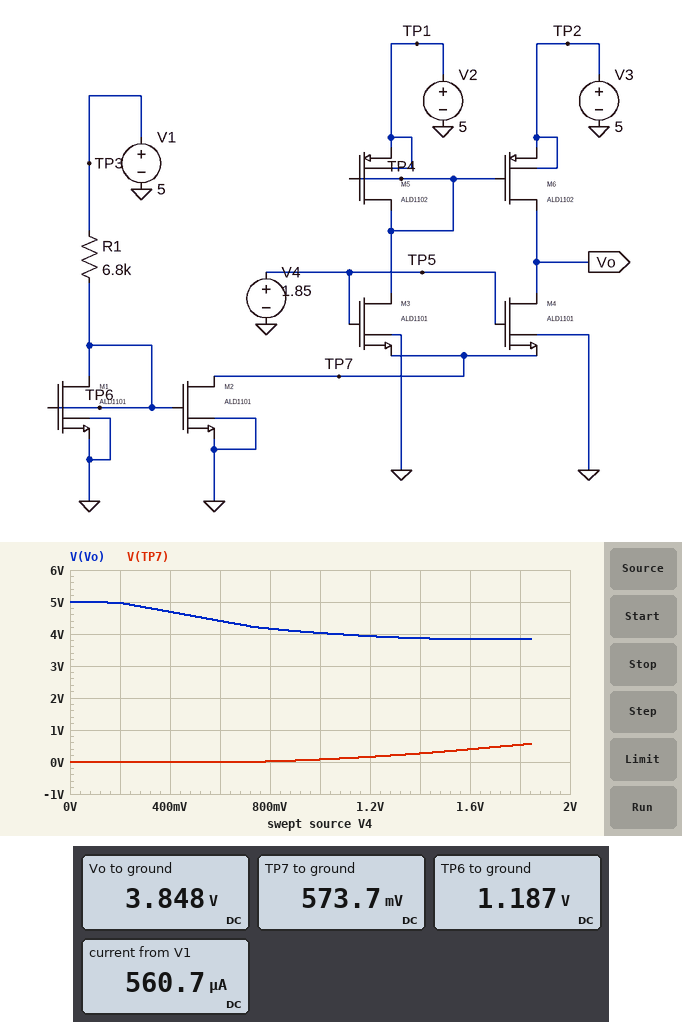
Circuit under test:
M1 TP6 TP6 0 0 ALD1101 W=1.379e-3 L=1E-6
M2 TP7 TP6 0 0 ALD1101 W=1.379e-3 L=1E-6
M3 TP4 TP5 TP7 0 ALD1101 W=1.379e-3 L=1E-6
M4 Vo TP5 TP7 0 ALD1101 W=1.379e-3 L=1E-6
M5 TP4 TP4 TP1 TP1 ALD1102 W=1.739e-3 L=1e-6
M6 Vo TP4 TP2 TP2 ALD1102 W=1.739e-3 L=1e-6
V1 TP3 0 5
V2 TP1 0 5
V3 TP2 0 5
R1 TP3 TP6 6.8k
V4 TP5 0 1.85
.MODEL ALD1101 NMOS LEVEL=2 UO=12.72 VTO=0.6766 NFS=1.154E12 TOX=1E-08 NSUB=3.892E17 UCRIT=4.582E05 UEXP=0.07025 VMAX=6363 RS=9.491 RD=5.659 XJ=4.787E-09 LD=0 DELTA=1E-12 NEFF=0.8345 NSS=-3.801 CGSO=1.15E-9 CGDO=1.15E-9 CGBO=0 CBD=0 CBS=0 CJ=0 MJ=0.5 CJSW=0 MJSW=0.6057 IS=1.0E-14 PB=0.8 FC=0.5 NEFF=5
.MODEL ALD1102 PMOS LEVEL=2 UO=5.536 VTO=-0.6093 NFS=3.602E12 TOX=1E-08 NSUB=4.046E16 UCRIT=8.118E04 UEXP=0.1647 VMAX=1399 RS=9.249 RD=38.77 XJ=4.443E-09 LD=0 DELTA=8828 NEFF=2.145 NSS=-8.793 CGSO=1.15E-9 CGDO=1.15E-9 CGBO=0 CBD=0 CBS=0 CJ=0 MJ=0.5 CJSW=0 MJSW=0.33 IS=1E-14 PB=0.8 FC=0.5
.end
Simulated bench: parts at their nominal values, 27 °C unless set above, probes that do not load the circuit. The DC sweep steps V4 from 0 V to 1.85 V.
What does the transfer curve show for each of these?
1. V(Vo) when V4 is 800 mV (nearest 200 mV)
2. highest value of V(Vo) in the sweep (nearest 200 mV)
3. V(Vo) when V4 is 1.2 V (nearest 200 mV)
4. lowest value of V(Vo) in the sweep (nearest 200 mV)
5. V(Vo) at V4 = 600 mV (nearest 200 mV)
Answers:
4.2 V
5.0 V
4.0 V
3.8 V
4.4 V
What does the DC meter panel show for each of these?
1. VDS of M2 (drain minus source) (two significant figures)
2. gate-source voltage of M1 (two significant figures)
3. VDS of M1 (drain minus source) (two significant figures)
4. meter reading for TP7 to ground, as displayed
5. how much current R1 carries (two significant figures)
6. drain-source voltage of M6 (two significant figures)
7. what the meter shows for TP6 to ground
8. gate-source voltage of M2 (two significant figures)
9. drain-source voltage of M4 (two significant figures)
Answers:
570 mV
1.2 V
1.2 V
573.7 mV
560 µA
-1.2 V
1.187 V
1.2 V
3.3 V
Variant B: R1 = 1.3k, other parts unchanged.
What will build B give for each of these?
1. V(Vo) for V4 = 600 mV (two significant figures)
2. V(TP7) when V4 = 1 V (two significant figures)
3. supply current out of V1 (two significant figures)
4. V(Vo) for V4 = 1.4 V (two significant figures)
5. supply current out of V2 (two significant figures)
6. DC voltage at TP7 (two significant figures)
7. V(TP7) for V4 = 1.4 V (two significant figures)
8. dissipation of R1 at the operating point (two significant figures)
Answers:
4.4 V
51 mV
2.5 mA
3.7 V
880 µA
370 mV
180 mV
8.0 mW
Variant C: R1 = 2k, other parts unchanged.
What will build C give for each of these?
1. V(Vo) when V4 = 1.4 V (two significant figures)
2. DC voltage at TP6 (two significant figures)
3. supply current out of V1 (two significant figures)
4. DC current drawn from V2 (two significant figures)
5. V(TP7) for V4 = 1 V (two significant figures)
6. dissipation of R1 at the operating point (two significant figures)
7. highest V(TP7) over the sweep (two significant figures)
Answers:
3.7 V
1.6 V
1.7 mA
730 µA
57 mV
5.8 mW
410 mV
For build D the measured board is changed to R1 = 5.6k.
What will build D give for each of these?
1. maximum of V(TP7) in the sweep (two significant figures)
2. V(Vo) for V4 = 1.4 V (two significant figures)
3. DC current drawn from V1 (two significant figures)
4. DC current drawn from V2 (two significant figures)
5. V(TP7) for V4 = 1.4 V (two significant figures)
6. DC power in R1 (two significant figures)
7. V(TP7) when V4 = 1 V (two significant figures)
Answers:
550 mV
3.8 V
670 µA
330 µA
250 mV
2.5 mW
75 mV
